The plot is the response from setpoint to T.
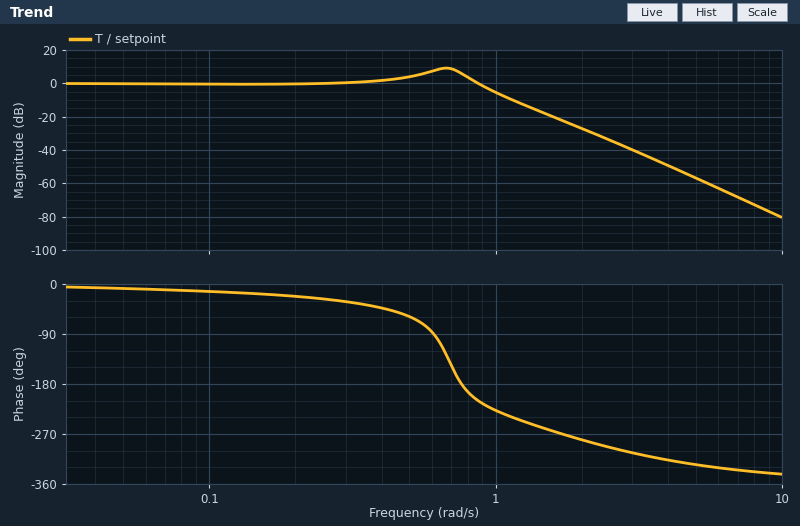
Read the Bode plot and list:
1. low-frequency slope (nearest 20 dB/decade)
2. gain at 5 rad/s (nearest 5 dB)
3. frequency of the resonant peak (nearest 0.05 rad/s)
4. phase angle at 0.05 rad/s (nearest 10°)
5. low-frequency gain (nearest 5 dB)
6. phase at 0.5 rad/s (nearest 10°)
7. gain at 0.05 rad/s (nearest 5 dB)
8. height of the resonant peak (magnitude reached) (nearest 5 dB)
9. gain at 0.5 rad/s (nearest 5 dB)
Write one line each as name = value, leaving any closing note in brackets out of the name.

low-frequency slope = 0 dB/decade
gain at 5 rad/s = -55 dB
frequency of the resonant peak = 0.65 rad/s
phase angle at 0.05 rad/s = -10°
low-frequency gain = 0 dB
phase at 0.5 rad/s = -60°
gain at 0.05 rad/s = 0 dB
height of the resonant peak (magnitude reached) = 10 dB
gain at 0.5 rad/s = 5 dB
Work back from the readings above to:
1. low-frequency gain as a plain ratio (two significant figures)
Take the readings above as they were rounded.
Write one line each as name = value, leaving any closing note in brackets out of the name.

low-frequency gain as a plain ratio = 1.0
